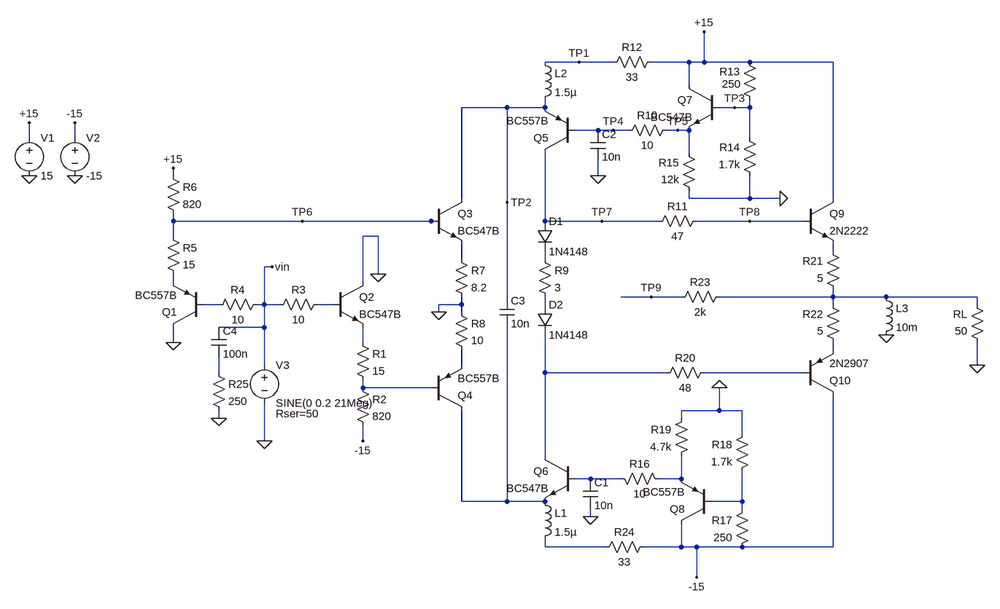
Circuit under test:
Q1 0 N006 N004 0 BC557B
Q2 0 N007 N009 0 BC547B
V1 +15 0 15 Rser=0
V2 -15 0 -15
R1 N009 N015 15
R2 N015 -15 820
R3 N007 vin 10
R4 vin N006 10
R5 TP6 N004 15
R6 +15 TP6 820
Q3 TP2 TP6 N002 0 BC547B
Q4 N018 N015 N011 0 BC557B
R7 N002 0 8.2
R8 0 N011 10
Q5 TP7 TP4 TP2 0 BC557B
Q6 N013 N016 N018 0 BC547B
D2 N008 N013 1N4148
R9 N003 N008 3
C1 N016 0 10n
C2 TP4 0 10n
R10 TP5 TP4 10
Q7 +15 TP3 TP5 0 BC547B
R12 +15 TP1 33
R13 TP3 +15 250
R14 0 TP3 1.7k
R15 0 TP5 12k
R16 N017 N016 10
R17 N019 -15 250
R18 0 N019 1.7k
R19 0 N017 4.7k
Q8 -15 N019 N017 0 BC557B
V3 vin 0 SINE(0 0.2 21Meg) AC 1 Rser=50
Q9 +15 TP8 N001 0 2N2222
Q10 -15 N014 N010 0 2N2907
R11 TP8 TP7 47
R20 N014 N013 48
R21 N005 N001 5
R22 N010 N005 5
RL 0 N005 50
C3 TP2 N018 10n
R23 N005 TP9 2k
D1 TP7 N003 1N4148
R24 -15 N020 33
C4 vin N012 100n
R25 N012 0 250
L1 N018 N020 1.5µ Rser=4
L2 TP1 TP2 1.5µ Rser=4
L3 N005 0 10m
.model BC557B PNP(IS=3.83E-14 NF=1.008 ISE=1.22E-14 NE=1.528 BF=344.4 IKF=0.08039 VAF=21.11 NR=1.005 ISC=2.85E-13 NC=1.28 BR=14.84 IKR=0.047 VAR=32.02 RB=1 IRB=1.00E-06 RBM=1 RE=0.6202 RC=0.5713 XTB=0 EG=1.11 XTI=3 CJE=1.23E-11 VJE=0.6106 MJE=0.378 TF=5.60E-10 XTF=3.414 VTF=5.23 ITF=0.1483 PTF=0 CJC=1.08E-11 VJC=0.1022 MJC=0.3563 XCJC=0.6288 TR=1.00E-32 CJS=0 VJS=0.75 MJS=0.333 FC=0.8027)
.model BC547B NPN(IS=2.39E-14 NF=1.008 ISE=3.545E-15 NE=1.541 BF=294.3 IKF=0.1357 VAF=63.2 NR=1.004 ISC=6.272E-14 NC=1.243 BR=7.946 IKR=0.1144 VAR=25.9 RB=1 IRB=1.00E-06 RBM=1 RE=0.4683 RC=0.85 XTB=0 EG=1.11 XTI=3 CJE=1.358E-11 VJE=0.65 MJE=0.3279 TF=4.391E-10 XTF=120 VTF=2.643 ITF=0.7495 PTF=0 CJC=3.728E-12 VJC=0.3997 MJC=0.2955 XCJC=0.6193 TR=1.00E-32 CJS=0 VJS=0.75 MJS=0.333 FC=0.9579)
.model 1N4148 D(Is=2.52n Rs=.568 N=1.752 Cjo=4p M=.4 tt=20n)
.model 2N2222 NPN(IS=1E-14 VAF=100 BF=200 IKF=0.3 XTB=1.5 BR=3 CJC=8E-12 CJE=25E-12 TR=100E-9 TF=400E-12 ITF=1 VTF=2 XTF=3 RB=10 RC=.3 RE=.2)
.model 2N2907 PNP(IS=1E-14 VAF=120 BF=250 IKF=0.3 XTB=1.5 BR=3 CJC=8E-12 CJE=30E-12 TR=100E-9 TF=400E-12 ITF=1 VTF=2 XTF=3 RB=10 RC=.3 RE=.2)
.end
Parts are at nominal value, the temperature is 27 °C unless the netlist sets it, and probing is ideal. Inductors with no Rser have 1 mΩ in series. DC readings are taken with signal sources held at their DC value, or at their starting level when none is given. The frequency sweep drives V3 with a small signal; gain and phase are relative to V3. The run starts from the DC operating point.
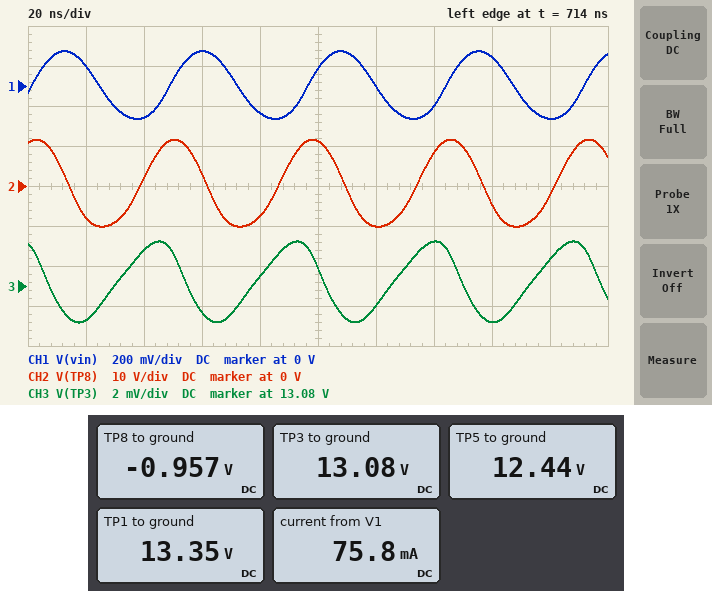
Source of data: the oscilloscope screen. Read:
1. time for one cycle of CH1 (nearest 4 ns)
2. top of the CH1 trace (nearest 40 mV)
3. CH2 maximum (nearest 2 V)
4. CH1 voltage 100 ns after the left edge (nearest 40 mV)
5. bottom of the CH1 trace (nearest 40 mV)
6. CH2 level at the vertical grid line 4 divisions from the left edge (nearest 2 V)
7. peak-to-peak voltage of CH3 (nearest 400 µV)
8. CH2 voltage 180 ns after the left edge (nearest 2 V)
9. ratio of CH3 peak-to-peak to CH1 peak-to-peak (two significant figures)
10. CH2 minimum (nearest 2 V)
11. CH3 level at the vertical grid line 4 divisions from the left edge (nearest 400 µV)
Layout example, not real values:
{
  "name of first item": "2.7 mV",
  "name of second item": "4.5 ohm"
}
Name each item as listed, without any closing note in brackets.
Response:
{
  "time for one cycle of CH1": "48 ns",
  "top of the CH1 trace": "160 mV",
  "CH2 maximum": "12 V",
  "CH1 voltage 100 ns after the left edge": "80 mV",
  "bottom of the CH1 trace": "-160 mV",
  "CH2 level at the vertical grid line 4 divisions from the left edge": "-8 V",
  "peak-to-peak voltage of CH3": "4.0 mV",
  "CH2 voltage 180 ns after the left edge": "-2 V",
  "ratio of CH3 peak-to-peak to CH1 peak-to-peak": "0.012",
  "CH2 minimum": "-10 V",
  "CH3 level at the vertical grid line 4 divisions from the left edge": "13.0764 V"
}
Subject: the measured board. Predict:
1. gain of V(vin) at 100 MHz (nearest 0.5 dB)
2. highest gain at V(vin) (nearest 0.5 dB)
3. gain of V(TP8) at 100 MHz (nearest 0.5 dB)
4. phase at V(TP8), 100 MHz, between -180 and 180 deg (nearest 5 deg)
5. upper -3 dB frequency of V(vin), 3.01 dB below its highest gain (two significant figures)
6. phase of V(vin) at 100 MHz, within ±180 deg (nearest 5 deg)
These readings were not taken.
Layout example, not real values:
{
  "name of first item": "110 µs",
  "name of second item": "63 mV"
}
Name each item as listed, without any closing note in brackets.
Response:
{
  "gain of V(vin) at 100 MHz": "-5.5 dB",
  "highest gain at V(vin)": "-0.5 dB",
  "gain of V(TP8) at 100 MHz": "15.0 dB",
  "phase at V(TP8), 100 MHz, between -180 and 180 deg": "-30 deg",
  "upper -3 dB frequency of V(vin), 3.01 dB below its highest gain": "85 MHz",
  "phase of V(vin) at 100 MHz, within ±180 deg": "-55 deg"
}
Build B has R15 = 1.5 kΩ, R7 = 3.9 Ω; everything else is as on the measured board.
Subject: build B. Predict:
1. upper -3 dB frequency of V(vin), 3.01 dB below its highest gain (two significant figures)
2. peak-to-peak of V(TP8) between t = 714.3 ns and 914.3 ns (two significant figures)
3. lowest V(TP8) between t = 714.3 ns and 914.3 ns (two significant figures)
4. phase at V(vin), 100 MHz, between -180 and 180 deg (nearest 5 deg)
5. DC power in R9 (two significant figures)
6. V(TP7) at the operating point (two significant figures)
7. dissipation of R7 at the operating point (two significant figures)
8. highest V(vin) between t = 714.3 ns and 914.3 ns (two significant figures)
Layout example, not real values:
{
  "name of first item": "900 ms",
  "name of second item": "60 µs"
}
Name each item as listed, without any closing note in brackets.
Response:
{
  "upper -3 dB frequency of V(vin), 3.01 dB below its highest gain": "74 MHz",
  "peak-to-peak of V(TP8) between t = 714.3 ns and 914.3 ns": "19 V",
  "lowest V(TP8) between t = 714.3 ns and 914.3 ns": "-12 V",
  "phase at V(vin), 100 MHz, between -180 and 180 deg": "-55 deg",
  "DC power in R9": "19 µW",
  "V(TP7) at the operating point": "-7.1 V",
  "dissipation of R7 at the operating point": "10 mW",
  "highest V(vin) between t = 714.3 ns and 914.3 ns": "180 mV"
}
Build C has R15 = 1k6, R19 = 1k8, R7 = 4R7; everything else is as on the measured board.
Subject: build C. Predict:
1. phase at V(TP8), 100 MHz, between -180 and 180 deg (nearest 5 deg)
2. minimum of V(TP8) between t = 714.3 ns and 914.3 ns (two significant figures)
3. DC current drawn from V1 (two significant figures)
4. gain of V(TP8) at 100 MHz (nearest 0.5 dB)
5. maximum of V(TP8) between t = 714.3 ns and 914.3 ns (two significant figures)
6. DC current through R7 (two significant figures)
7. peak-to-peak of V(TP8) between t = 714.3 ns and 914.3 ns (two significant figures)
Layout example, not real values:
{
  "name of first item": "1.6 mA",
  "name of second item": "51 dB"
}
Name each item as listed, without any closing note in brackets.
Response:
{
  "phase at V(TP8), 100 MHz, between -180 and 180 deg": "-25 deg",
  "minimum of V(TP8) between t = 714.3 ns and 914.3 ns": "-12 V",
  "DC current drawn from V1": "85 mA",
  "gain of V(TP8) at 100 MHz": "13.0 dB",
  "maximum of V(TP8) between t = 714.3 ns and 914.3 ns": "6.5 V",
  "DC current through R7": "45 mA",
  "peak-to-peak of V(TP8) between t = 714.3 ns and 914.3 ns": "18 V"
}
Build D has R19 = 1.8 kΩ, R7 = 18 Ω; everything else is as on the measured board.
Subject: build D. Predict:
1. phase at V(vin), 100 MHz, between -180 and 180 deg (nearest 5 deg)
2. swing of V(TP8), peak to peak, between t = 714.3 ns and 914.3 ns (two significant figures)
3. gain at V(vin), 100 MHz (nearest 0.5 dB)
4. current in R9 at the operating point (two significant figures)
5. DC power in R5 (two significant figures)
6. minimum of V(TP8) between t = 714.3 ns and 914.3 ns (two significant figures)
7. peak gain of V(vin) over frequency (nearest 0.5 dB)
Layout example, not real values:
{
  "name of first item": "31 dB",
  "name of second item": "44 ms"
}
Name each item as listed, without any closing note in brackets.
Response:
{
  "phase at V(vin), 100 MHz, between -180 and 180 deg": "-50 deg",
  "swing of V(TP8), peak to peak, between t = 714.3 ns and 914.3 ns": "12 V",
  "gain at V(vin), 100 MHz": "-4.5 dB",
  "current in R9 at the operating point": "25 mA",
  "DC power in R5": "4.4 mW",
  "minimum of V(TP8) between t = 714.3 ns and 914.3 ns": "-2.6 V",
  "peak gain of V(vin) over frequency": "-1.0 dB"
}
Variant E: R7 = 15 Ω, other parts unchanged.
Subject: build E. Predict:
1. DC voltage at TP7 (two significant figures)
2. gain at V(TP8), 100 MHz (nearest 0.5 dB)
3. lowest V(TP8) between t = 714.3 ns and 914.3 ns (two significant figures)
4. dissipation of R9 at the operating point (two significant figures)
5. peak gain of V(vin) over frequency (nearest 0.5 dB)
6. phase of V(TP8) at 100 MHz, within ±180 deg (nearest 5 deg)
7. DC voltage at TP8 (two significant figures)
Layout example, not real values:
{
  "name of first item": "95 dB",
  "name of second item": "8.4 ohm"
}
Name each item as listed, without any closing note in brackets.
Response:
{
  "DC voltage at TP7": "4.7 V",
  "gain at V(TP8), 100 MHz": "11.5 dB",
  "lowest V(TP8) between t = 714.3 ns and 914.3 ns": "-3.9 V",
  "dissipation of R9 at the operating point": "1.7 mW",
  "peak gain of V(vin) over frequency": "-1.0 dB",
  "phase of V(TP8) at 100 MHz, within ±180 deg": "-25 deg",
  "DC voltage at TP8": "4.3 V"
}
